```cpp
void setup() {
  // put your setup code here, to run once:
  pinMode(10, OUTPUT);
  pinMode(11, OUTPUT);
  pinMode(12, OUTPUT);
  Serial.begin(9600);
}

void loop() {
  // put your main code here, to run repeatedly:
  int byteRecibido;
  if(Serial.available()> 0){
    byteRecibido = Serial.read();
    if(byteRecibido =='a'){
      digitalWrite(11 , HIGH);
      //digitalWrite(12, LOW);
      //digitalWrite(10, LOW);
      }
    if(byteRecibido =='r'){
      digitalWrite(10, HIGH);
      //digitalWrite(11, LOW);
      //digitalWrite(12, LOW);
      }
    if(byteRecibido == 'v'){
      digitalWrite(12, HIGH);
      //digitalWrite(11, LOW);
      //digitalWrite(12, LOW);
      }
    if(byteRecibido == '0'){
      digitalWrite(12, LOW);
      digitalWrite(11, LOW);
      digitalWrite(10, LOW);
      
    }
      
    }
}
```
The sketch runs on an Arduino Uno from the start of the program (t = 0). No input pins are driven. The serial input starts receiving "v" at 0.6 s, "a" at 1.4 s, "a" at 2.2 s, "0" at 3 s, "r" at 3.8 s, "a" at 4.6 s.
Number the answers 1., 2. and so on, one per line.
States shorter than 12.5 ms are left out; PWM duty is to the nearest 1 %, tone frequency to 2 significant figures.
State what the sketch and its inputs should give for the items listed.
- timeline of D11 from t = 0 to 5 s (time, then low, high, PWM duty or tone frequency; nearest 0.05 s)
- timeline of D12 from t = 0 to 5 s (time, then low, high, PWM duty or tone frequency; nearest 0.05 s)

1. 0 s low; 1.4 s high; 3 s low; 4.6 s high
2. 0 s low; 0.6 s high; 3 s low
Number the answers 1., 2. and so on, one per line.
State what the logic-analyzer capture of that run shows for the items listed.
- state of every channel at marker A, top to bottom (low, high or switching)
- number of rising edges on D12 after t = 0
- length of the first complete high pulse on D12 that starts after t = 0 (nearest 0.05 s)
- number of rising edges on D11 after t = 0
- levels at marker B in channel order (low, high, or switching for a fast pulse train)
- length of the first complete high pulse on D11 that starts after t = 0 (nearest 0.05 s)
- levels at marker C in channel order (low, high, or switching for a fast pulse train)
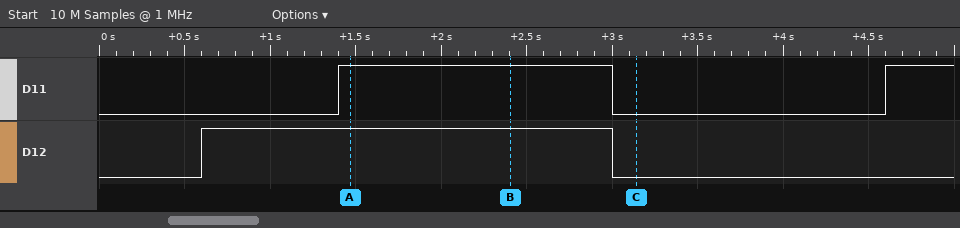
1. D11 high, D12 high
2. 1
3. 2.40 s
4. 2
5. D11 high, D12 high
6. 1.60 s
7. D11 low, D12 low
